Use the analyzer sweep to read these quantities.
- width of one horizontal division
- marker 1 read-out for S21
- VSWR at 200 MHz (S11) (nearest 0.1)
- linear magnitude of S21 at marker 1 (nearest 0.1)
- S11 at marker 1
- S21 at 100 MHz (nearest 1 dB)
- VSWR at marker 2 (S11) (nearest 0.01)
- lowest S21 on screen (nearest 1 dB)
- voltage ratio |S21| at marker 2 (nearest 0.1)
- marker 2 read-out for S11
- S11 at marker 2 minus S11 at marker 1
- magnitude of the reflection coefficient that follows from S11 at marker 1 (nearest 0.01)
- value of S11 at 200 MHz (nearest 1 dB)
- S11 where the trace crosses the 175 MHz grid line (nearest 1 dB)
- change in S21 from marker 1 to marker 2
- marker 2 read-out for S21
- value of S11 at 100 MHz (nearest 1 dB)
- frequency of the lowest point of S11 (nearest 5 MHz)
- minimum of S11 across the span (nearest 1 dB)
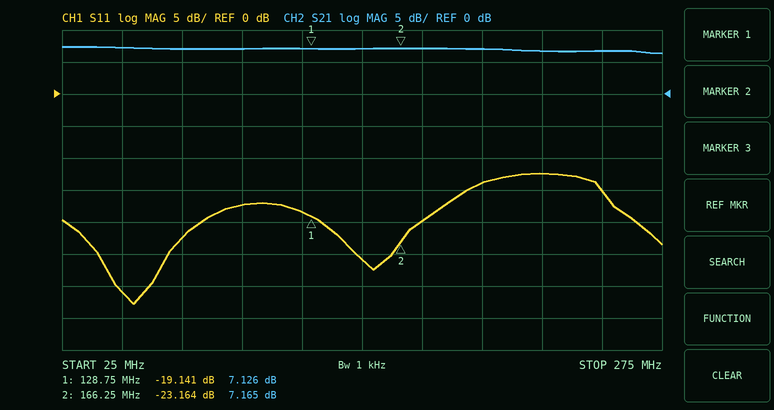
25 MHz
7.126 dB
1.5
2.3
-19.141 dB
7 dB
1.15
6 dB
2.3
-23.164 dB
-4.023 dB
0.11
-14 dB
-20 dB
0.039 dB
7.165 dB
-17 dB
55 MHz
-33 dB
